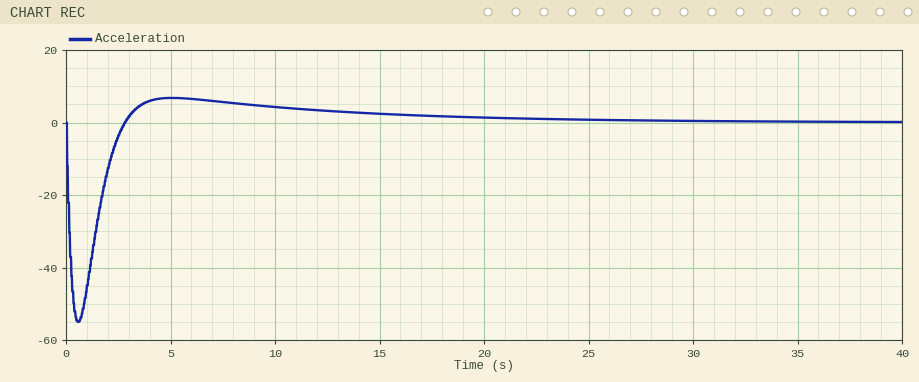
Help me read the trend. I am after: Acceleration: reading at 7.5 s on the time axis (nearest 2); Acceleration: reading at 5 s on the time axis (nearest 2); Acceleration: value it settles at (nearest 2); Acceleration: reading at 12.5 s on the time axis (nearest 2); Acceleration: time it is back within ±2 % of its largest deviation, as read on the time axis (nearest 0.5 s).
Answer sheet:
6
6
0
4
22.0 s
